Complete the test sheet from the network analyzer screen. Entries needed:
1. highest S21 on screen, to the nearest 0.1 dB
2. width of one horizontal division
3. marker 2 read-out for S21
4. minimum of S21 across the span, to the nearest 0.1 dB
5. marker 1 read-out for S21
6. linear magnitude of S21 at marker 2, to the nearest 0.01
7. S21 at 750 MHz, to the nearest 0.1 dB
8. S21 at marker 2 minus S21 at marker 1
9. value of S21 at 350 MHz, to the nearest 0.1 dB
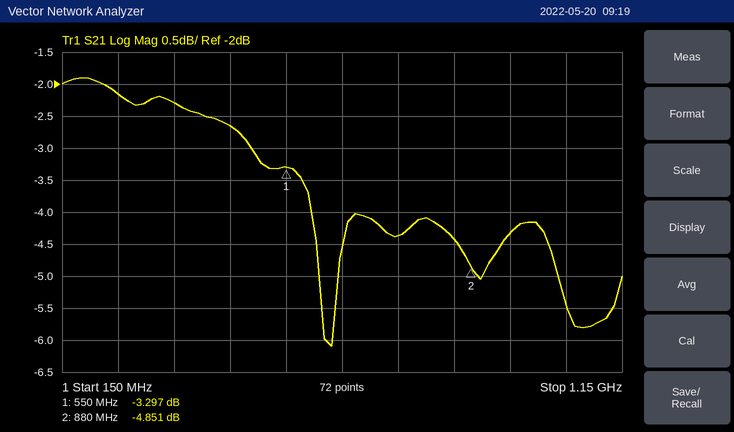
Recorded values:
-1.9 dB
100 MHz
-4.851 dB
-6.1 dB
-3.297 dB
0.57
-4.4 dB
-1.554 dB
-2.3 dB
